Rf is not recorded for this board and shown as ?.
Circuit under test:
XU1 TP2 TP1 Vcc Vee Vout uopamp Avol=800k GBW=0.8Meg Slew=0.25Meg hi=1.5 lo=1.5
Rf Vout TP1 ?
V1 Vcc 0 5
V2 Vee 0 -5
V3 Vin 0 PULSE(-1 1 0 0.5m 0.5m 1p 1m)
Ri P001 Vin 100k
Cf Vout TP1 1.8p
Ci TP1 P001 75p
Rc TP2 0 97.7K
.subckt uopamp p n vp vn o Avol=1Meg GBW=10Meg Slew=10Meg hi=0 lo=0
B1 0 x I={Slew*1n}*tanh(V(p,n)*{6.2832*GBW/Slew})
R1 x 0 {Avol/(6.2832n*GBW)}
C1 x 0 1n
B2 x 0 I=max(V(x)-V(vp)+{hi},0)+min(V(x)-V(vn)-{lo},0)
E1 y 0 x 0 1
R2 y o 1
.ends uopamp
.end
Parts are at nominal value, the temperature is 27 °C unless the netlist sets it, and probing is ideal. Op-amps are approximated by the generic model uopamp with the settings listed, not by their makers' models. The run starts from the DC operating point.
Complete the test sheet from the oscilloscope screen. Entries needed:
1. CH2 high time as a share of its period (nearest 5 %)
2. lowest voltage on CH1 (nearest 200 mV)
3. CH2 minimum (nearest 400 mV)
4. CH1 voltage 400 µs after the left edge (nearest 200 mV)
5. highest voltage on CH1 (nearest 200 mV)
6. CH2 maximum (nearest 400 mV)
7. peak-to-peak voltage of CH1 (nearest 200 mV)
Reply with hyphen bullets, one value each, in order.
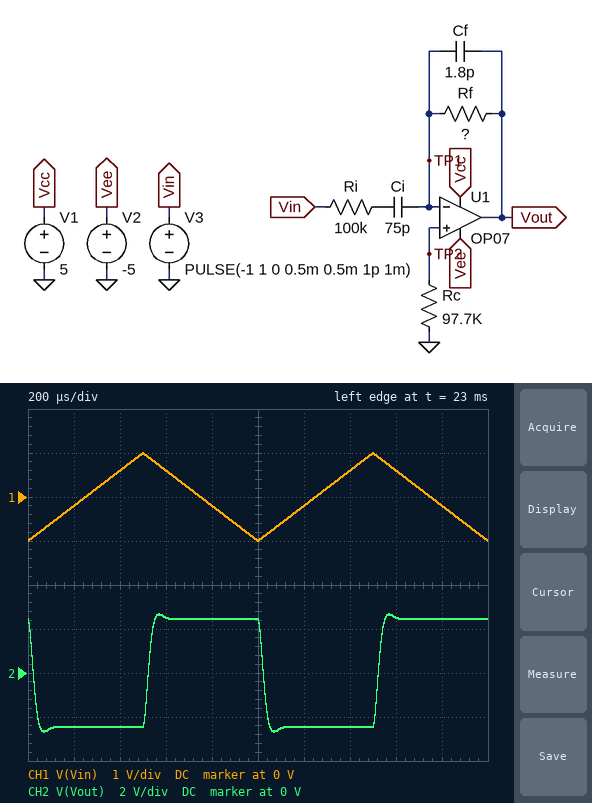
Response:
- 50 %
- -1.0 V
- -2.8 V
- 600 mV
- 1.0 V
- 2.8 V
- 2.0 V
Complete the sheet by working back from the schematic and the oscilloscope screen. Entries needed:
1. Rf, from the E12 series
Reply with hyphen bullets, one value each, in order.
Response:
- 8.2 MΩ
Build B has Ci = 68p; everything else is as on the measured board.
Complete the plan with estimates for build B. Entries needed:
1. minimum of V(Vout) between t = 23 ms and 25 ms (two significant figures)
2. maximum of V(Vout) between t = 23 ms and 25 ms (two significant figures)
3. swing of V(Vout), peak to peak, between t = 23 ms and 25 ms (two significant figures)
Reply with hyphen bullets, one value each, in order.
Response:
- -2.4 V
- 2.4 V
- 4.8 V
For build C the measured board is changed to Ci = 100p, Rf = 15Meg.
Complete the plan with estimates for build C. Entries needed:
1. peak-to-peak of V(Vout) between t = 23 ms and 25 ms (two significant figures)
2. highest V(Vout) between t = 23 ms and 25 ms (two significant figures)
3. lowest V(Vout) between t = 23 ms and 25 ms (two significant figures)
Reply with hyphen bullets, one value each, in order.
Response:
- 7.0 V
- 3.5 V
- -3.5 V
